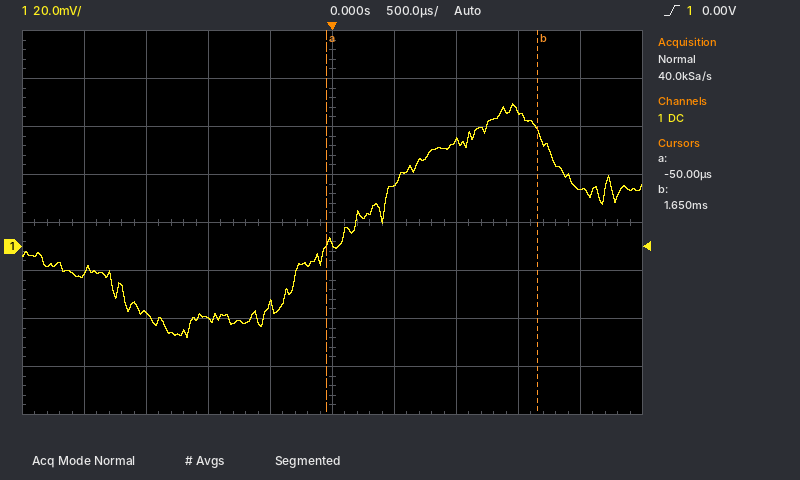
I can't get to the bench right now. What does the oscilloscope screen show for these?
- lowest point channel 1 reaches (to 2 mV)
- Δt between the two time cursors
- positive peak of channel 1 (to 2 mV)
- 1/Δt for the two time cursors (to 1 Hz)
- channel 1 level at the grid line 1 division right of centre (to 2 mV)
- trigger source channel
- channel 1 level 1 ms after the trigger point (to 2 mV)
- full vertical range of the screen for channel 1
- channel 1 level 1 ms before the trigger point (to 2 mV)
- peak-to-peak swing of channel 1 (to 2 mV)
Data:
-38 mV
1.70 ms
60 mV
588 Hz
26 mV
channel 1
44 mV
160 mV
-30 mV
98 mV
